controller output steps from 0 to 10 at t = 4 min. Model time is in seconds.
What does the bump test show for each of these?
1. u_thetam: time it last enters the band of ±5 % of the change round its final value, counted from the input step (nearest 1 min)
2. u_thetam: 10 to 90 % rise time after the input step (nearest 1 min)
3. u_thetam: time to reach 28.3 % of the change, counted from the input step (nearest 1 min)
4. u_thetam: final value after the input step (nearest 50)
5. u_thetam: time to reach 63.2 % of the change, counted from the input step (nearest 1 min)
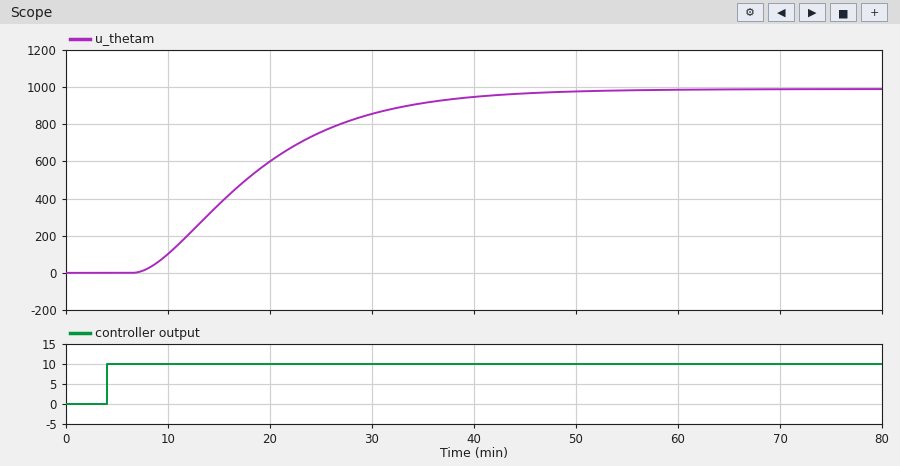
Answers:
35 min
23 min
9 min
1000
17 min
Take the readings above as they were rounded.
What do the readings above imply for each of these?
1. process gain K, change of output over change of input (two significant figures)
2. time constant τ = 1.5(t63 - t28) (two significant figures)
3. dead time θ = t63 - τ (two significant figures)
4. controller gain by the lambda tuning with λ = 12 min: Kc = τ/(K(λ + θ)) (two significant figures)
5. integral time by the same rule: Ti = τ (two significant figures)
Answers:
100
12 min
5.0 min
0.0071
12 min
